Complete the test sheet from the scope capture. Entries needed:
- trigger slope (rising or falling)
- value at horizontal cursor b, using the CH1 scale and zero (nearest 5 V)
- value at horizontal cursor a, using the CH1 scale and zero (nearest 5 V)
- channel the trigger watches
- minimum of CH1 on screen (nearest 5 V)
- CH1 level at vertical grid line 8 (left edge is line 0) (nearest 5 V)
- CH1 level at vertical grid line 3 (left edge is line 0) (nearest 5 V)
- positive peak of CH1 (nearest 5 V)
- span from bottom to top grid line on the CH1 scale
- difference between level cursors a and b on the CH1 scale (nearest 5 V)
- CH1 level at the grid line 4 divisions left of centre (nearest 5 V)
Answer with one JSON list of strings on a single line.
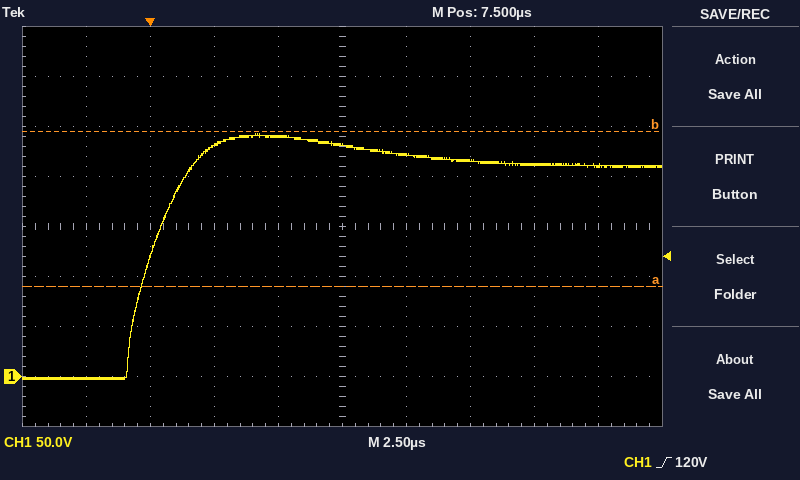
["rising", "245 V", "90 V", "CH1", "-5 V", "210 V", "230 V", "245 V", "400 V", "155 V", "0 V"]
